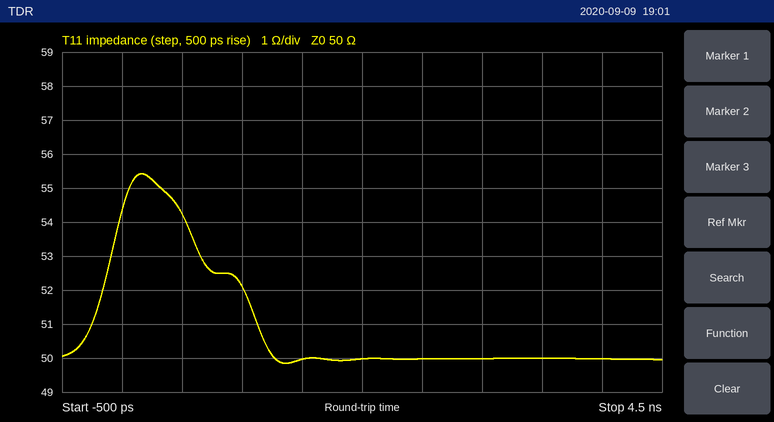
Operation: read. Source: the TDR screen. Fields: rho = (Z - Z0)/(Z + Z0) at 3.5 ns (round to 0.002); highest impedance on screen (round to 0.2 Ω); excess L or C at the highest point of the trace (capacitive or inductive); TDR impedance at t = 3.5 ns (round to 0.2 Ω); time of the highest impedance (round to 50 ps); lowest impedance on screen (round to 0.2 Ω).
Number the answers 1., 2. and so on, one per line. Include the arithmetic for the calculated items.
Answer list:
1. (50 − 50)/(50 + 50) ≈ 0.000
2. 55.4 Ω
3. inductive
4. 50.0 Ω
5. 150 ps
6. 49.8 Ω
